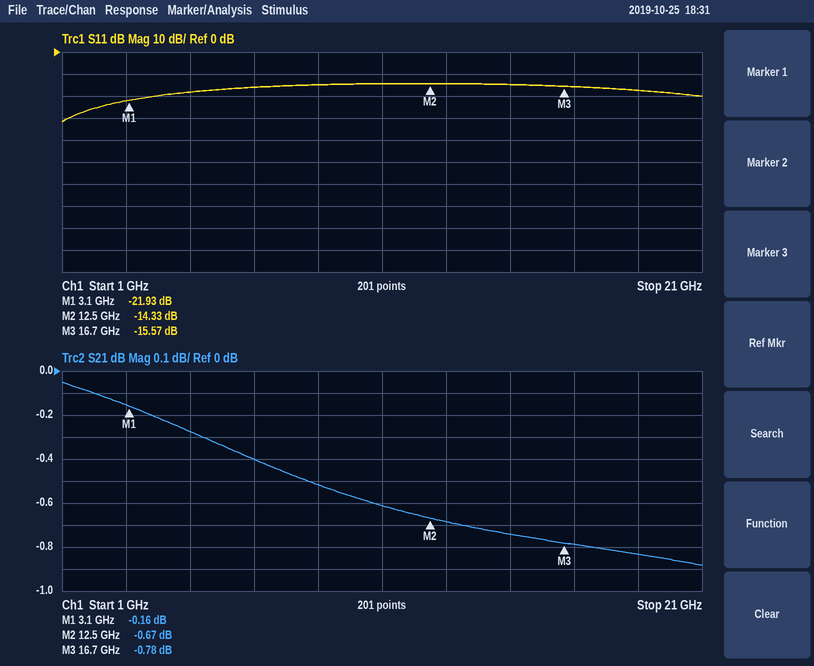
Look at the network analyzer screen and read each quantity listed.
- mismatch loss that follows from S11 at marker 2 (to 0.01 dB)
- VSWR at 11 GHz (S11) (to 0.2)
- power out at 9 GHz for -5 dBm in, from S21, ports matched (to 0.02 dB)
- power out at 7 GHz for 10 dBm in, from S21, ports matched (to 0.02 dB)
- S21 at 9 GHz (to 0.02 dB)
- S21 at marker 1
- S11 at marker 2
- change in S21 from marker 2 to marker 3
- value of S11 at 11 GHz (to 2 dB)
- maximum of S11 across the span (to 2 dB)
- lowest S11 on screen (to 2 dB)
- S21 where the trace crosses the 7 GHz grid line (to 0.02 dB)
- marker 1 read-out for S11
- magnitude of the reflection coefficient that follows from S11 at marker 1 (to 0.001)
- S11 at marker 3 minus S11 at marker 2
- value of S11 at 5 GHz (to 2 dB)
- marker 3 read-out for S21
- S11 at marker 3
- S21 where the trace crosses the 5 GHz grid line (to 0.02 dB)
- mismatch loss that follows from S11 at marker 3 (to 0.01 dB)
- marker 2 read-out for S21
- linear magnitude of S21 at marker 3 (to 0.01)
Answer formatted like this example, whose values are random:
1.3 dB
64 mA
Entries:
0.16 dB
1.4
-5.52 dBm
9.60 dBm
-0.52 dB
-0.16 dB
-14.33 dB
-0.11 dB
-14 dB
-14 dB
-32 dB
-0.40 dB
-21.93 dB
0.080
-1.24 dB
-18 dB
-0.78 dB
-15.57 dB
-0.28 dB
0.12 dB
-0.67 dB
0.91
